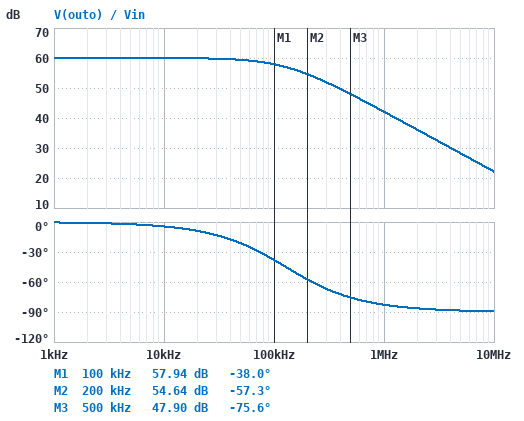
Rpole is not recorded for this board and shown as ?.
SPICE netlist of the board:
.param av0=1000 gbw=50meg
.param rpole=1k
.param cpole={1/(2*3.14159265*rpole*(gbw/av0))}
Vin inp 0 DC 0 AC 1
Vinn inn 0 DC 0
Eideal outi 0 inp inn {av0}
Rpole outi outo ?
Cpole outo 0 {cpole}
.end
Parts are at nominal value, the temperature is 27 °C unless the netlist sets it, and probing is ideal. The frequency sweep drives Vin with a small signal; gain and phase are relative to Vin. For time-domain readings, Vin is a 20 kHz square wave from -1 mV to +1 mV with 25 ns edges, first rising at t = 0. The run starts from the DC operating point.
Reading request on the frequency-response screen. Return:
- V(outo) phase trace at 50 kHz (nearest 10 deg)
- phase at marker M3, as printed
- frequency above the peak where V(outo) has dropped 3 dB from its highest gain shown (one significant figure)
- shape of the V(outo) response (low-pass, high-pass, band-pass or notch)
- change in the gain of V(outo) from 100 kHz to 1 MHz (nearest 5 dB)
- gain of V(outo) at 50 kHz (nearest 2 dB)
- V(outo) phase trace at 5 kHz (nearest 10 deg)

-20 deg
-75.6 deg
100 kHz
low-pass
-15 dB
60 dB
0 deg
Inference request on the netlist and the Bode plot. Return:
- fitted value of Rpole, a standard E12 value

390 Ω
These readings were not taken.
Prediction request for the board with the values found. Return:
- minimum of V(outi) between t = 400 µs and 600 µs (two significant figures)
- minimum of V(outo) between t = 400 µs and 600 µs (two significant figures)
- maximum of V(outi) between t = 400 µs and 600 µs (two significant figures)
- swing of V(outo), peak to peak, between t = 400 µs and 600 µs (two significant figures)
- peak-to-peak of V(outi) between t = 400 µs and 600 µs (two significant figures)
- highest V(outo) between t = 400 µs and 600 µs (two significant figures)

-1.0 V
-1.0 V
1.0 V
2.0 V
2.0 V
1.0 V
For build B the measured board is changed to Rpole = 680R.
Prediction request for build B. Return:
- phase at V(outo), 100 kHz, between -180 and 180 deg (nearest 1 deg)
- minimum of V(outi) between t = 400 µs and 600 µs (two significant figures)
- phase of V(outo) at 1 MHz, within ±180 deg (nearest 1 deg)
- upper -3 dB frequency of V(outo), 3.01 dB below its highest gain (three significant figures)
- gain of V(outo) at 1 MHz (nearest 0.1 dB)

-54 deg
-1.0 V
-86 deg
73.5 kHz
37.3 dB
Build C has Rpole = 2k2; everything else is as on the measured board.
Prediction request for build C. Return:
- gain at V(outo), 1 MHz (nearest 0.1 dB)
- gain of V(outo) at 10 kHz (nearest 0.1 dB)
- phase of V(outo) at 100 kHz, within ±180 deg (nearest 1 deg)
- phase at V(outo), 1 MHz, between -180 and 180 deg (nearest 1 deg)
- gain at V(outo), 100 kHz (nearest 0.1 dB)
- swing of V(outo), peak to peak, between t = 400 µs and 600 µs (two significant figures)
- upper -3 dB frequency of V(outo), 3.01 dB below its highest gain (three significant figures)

27.1 dB
59.2 dB
-77 deg
-89 deg
46.9 dB
1.9 V
22.7 kHz
